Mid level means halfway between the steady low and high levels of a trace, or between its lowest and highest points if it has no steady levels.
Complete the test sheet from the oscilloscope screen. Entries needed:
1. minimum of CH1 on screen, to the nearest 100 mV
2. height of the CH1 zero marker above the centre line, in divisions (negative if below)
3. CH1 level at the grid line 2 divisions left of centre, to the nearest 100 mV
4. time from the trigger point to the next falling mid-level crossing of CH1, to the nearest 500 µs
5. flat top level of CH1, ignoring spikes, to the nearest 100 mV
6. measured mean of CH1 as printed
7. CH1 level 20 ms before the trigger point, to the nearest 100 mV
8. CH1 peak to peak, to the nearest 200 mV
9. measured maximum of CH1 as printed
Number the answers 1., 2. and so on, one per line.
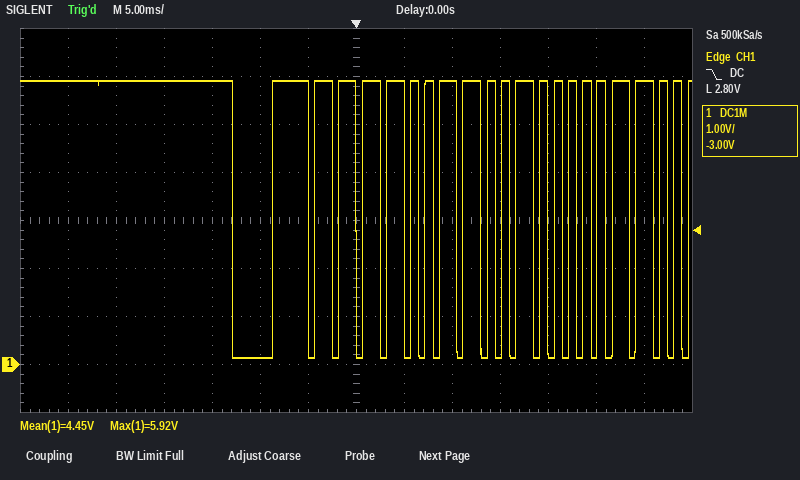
1. 100 mV
2. -3.0 div
3. 100 mV
4. 2.5 ms
5. 5.9 V
6. 4.45 V
7. 5.9 V
8. 5.8 V
9. 5.92 V
